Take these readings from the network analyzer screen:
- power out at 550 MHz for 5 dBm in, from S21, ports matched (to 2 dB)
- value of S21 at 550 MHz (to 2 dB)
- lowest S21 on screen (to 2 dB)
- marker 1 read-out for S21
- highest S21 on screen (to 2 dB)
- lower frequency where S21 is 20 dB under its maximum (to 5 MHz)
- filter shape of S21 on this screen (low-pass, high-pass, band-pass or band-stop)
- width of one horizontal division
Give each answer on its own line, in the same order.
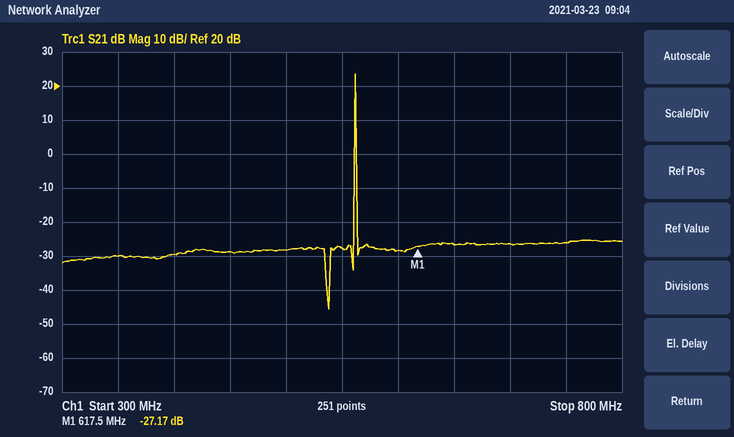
-22 dBm
-28 dB
-46 dB
-27.17 dB
24 dB
560 MHz
band-pass
50 MHz
